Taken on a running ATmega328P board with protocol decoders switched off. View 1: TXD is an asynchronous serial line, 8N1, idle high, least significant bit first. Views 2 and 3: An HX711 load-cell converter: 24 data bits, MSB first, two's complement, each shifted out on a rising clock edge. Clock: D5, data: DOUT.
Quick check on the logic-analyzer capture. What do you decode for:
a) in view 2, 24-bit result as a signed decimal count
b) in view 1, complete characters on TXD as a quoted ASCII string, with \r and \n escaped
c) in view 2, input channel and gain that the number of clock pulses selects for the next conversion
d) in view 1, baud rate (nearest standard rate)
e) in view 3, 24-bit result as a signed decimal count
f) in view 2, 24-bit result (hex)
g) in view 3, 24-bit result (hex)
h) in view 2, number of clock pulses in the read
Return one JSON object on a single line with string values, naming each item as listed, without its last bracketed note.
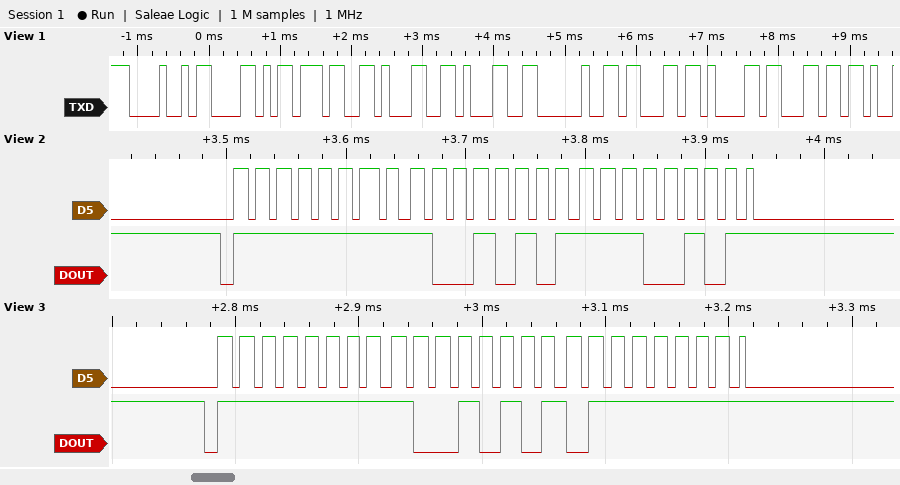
{"in view 2, 24-bit result as a signed decimal count": "-27163", "in view 1, complete characters on TXD as a quoted ASCII string, with \\r and \\n escaped": "\"HX711 cal\"", "in view 2, input channel and gain that the number of clock pulses selects for the next conversion": "channel A, gain 128", "in view 1, baud rate": "9600 baud", "in view 3, 24-bit result as a signed decimal count": "-27265", "in view 2, 24-bit result": "0xFF95E5", "in view 3, 24-bit result": "0xFF957F", "in view 2, number of clock pulses in the read": "25"}
